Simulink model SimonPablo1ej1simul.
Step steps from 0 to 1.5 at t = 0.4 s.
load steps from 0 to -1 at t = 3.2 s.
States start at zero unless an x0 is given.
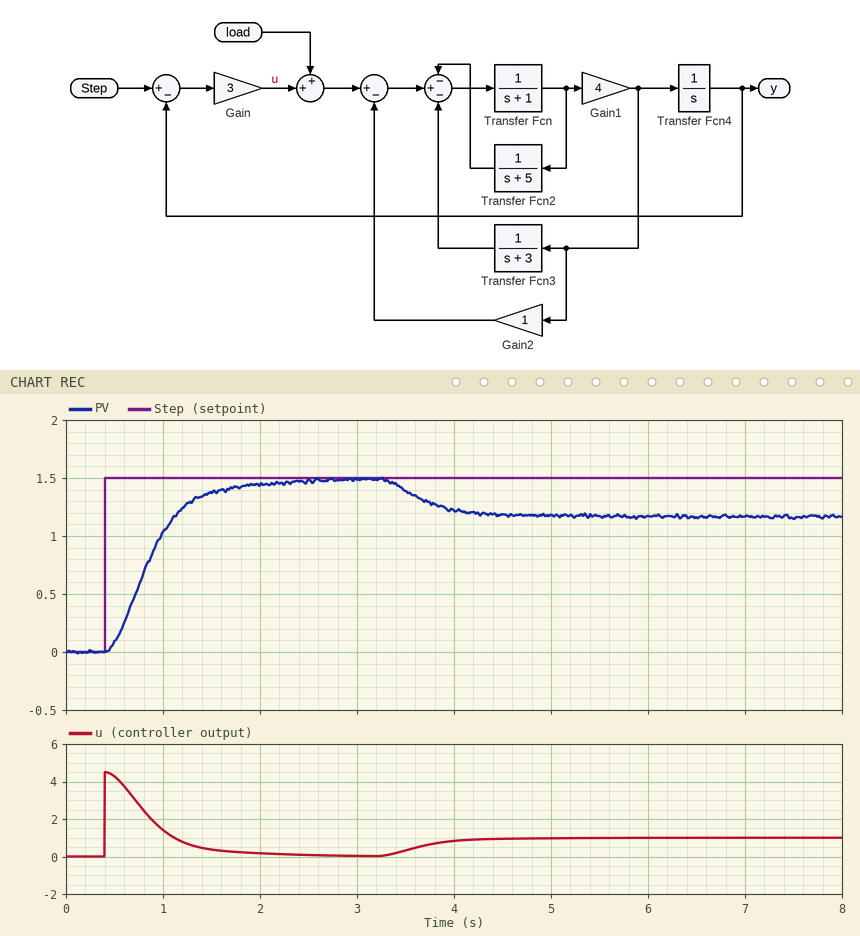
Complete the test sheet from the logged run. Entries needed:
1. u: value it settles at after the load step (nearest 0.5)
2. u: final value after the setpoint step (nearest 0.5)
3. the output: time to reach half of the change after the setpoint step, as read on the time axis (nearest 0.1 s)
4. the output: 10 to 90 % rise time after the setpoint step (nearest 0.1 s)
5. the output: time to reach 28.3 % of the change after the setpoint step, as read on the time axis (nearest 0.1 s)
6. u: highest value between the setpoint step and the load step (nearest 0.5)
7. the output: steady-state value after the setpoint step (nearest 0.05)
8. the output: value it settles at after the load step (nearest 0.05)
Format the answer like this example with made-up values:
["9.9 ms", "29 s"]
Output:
["1.0", "0.0", "0.8 s", "0.9 s", "0.7 s", "4.5", "1.50", "1.15"]
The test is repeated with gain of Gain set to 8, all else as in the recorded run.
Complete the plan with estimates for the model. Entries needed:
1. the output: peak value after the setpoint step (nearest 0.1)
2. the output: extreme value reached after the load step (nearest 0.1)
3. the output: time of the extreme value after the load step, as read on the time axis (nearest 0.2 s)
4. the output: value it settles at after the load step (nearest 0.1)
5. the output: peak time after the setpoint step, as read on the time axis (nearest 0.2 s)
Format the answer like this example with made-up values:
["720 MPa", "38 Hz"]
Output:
["1.7", "1.4", "3.8 s", "1.4", "1.0 s"]
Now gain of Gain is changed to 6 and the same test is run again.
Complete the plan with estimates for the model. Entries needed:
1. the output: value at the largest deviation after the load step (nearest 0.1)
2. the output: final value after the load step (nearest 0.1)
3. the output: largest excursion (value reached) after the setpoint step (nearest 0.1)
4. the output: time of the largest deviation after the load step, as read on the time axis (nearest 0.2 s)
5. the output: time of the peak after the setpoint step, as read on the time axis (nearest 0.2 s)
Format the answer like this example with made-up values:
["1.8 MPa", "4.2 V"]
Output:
["1.3", "1.3", "1.6", "4.0 s", "1.2 s"]
